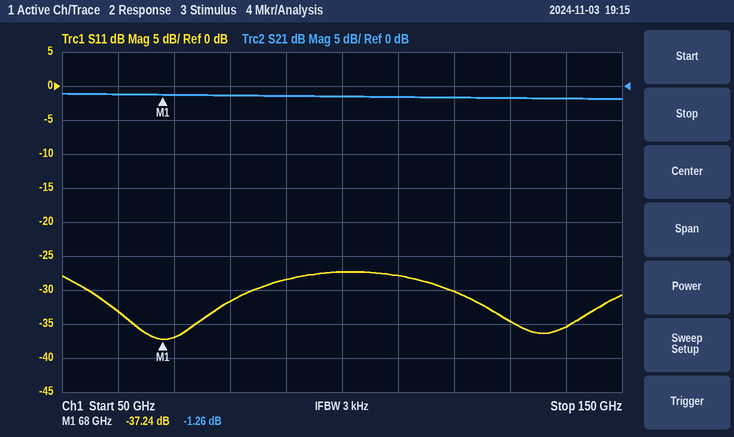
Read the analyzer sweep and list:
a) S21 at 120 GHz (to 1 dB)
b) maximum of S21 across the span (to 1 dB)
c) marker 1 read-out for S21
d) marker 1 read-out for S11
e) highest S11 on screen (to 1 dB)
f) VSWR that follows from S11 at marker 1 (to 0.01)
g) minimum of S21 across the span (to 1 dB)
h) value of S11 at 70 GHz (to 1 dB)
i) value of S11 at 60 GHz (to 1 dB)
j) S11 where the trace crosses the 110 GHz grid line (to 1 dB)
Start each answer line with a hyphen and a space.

- -2 dB
- -1 dB
- -1.26 dB
- -37.24 dB
- -27 dB
- 1.03
- -2 dB
- -37 dB
- -33 dB
- -28 dB
